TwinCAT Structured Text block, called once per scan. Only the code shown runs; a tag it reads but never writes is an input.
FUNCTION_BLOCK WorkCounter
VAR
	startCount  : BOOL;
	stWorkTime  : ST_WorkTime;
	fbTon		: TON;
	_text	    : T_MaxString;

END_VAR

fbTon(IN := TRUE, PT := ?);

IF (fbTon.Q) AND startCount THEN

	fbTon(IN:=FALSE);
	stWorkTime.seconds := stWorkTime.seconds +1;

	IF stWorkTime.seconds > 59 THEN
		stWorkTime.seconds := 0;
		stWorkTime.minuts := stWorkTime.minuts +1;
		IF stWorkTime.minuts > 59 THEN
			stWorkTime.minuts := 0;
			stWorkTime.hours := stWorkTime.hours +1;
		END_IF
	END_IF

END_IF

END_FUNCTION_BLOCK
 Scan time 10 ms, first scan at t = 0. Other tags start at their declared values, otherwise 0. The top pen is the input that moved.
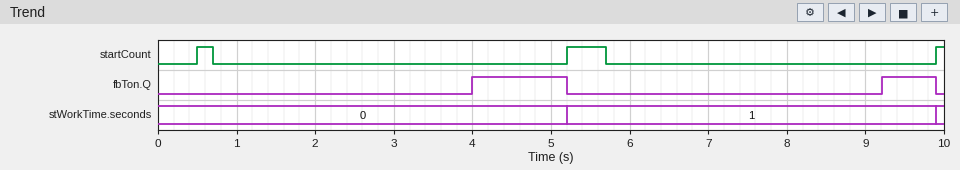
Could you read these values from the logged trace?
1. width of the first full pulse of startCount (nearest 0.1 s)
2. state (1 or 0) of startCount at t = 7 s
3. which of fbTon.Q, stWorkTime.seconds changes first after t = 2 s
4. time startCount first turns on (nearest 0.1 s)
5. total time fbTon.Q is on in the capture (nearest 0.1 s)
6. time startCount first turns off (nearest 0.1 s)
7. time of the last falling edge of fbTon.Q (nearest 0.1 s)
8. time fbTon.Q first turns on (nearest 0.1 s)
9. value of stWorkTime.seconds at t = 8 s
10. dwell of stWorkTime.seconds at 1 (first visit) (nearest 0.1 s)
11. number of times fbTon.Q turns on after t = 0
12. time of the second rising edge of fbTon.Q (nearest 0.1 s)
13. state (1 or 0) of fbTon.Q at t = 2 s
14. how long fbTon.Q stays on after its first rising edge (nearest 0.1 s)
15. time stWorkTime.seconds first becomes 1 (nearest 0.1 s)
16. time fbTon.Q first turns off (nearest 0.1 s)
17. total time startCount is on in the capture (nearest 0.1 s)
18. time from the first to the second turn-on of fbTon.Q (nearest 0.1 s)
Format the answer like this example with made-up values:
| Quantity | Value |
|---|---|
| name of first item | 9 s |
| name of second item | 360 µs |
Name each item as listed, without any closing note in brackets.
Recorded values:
| Quantity | Value |
|---|---|
| width of the first full pulse of startCount | 0.2 s |
| state (1 or 0) of startCount at t = 7 s | 0 |
| which of fbTon.Q, stWorkTime.seconds changes first after t = 2 s | fbTon.Q |
| time startCount first turns on | 0.5 s |
| total time fbTon.Q is on in the capture | 1.9 s |
| time startCount first turns off | 0.7 s |
| time of the last falling edge of fbTon.Q | 9.9 s |
| time fbTon.Q first turns on | 4.0 s |
| value of stWorkTime.seconds at t = 8 s | 1 |
| dwell of stWorkTime.seconds at 1 (first visit) | 4.7 s |
| number of times fbTon.Q turns on after t = 0 | 2 |
| time of the second rising edge of fbTon.Q | 9.2 s |
| state (1 or 0) of fbTon.Q at t = 2 s | 0 |
| how long fbTon.Q stays on after its first rising edge | 1.2 s |
| time stWorkTime.seconds first becomes 1 | 5.2 s |
| time fbTon.Q first turns off | 5.2 s |
| total time startCount is on in the capture | 0.8 s |
| time from the first to the second turn-on of fbTon.Q | 5.2 s |
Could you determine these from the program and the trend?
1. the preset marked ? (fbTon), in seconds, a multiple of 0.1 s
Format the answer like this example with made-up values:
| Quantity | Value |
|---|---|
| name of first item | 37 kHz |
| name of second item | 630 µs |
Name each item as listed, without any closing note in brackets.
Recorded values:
| Quantity | Value |
|---|---|
| the preset marked ? (fbTon), in seconds, a multiple of 0.1 s | 4.0 s |
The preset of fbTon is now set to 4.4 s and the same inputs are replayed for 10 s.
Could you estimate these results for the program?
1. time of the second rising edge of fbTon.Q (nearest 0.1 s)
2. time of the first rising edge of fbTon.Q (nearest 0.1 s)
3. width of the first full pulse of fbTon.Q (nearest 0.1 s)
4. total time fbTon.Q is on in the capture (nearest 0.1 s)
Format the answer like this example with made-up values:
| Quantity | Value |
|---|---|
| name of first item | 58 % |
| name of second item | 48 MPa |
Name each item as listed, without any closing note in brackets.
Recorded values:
| Quantity | Value |
|---|---|
| time of the second rising edge of fbTon.Q | 9.6 s |
| time of the first rising edge of fbTon.Q | 4.4 s |
| width of the first full pulse of fbTon.Q | 0.8 s |
| total time fbTon.Q is on in the capture | 1.1 s |
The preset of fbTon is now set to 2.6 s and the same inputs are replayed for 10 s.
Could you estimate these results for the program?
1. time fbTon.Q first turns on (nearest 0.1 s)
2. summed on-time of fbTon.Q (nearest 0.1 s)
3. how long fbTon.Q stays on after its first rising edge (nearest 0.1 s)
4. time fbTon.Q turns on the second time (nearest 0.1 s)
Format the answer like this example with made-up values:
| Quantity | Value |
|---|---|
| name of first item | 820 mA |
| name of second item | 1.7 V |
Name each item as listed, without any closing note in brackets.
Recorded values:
| Quantity | Value |
|---|---|
| time fbTon.Q first turns on | 2.6 s |
| summed on-time of fbTon.Q | 4.7 s |
| how long fbTon.Q stays on after its first rising edge | 2.6 s |
| time fbTon.Q turns on the second time | 7.8 s |
